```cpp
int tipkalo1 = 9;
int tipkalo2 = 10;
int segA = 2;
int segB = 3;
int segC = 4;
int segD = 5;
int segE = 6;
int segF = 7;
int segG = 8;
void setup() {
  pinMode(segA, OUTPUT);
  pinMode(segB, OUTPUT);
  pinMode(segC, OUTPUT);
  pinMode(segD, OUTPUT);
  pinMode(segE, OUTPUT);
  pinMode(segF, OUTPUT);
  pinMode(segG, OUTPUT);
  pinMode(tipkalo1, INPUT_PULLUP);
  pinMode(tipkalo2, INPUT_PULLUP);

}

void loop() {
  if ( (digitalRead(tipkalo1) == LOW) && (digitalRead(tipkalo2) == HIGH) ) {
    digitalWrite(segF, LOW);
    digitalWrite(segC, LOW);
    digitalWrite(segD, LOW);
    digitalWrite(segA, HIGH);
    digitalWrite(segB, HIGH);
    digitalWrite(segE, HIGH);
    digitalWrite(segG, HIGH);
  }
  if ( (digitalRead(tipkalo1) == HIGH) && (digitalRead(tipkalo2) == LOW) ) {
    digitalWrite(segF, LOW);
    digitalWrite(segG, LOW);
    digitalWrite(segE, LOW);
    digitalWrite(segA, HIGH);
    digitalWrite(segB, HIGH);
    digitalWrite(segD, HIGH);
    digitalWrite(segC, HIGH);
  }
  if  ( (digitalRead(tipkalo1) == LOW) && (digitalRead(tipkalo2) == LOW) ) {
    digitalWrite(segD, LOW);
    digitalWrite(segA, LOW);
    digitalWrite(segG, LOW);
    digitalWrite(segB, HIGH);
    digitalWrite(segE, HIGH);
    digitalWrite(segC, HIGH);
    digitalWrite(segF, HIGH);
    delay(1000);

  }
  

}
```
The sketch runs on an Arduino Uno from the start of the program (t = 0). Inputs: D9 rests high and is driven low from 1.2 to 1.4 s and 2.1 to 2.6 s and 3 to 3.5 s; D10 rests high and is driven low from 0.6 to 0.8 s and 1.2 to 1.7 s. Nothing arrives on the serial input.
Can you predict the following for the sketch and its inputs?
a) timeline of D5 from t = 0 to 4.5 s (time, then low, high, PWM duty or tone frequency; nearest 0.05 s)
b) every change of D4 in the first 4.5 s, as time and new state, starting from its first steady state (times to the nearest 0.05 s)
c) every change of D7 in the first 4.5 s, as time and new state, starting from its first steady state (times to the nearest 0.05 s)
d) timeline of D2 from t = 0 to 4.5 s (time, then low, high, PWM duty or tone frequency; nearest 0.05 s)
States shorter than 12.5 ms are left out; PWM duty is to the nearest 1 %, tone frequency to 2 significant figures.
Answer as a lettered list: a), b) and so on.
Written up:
a) 0 s low; 0.6 s high; 1.2 s low
b) 0 s low; 0.6 s high; 2.2 s low
c) 0 s low; 1.2 s high; 2.2 s low
d) 0 s low; 0.6 s high; 1.2 s low; 2.2 s high
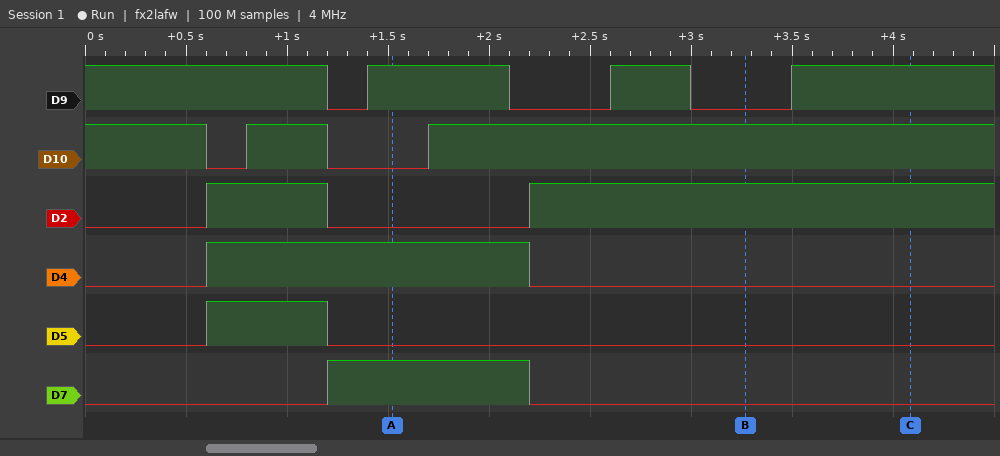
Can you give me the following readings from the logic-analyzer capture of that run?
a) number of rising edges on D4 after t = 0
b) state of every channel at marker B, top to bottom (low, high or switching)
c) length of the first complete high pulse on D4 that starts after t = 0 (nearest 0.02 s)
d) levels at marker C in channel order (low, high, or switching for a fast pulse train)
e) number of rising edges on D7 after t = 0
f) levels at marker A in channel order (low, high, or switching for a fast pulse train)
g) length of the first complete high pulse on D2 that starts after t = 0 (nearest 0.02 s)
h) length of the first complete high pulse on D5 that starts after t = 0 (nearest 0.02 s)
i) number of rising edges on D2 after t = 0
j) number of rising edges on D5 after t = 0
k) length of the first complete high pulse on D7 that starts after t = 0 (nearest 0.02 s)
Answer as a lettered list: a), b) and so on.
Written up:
a) 1
b) D9 low, D10 high, D2 high, D4 low, D5 low, D7 low
c) 1.60 s
d) D9 high, D10 high, D2 high, D4 low, D5 low, D7 low
e) 1
f) D9 high, D10 low, D2 low, D4 high, D5 low, D7 high
g) 0.60 s
h) 0.60 s
i) 2
j) 1
k) 1.00 s
